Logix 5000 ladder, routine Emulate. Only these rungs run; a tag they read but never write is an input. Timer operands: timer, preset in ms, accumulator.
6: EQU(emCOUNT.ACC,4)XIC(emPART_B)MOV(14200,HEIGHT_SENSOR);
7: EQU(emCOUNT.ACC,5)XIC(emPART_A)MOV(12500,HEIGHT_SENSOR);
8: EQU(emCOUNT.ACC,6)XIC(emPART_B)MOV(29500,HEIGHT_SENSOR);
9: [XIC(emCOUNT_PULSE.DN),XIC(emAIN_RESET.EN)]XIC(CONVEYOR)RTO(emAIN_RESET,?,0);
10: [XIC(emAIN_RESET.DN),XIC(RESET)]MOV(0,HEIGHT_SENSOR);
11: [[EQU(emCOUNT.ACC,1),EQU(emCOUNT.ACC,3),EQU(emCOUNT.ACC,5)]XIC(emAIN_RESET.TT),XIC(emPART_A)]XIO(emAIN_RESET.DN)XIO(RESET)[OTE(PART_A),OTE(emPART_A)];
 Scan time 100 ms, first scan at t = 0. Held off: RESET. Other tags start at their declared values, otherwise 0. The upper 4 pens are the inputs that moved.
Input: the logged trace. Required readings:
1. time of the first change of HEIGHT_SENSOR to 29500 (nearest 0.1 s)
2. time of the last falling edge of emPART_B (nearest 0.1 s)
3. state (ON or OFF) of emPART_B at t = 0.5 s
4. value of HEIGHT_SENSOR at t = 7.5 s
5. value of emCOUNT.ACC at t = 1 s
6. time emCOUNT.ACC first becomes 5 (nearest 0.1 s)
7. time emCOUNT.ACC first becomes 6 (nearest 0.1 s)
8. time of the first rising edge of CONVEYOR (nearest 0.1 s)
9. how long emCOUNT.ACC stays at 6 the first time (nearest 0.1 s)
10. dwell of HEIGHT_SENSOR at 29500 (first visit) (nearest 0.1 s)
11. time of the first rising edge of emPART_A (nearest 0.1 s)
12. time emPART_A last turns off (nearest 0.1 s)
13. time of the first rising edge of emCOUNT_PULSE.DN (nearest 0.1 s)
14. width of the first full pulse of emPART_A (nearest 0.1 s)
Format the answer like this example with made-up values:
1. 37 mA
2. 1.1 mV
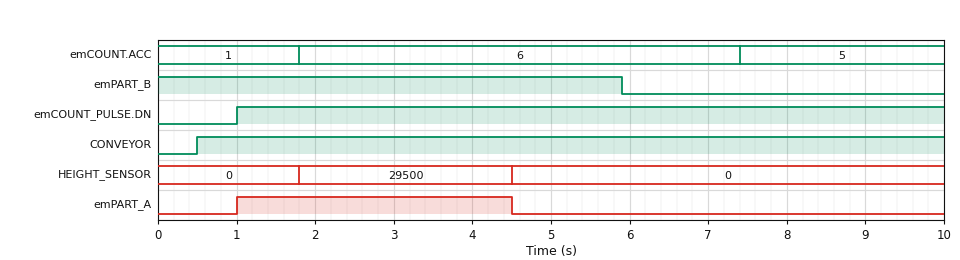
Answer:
1. 1.8 s
2. 5.9 s
3. ON
4. 0
5. 1
6. 7.4 s
7. 1.8 s
8. 0.5 s
9. 5.6 s
10. 2.7 s
11. 1.0 s
12. 4.5 s
13. 1.0 s
14. 3.5 s
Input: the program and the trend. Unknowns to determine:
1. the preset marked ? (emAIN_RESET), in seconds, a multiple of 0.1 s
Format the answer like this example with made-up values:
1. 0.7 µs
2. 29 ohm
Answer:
1. 3.5 s
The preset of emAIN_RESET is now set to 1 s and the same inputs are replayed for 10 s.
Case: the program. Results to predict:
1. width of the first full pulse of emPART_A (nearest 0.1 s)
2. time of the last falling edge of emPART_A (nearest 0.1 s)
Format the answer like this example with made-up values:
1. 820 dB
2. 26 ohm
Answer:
1. 1.0 s
2. 2.0 s
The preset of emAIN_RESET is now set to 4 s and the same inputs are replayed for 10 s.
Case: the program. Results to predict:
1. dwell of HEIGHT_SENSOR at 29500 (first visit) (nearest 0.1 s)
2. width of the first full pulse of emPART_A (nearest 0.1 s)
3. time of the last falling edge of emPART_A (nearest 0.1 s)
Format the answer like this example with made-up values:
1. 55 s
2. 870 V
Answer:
1. 3.2 s
2. 4.0 s
3. 5.0 s
